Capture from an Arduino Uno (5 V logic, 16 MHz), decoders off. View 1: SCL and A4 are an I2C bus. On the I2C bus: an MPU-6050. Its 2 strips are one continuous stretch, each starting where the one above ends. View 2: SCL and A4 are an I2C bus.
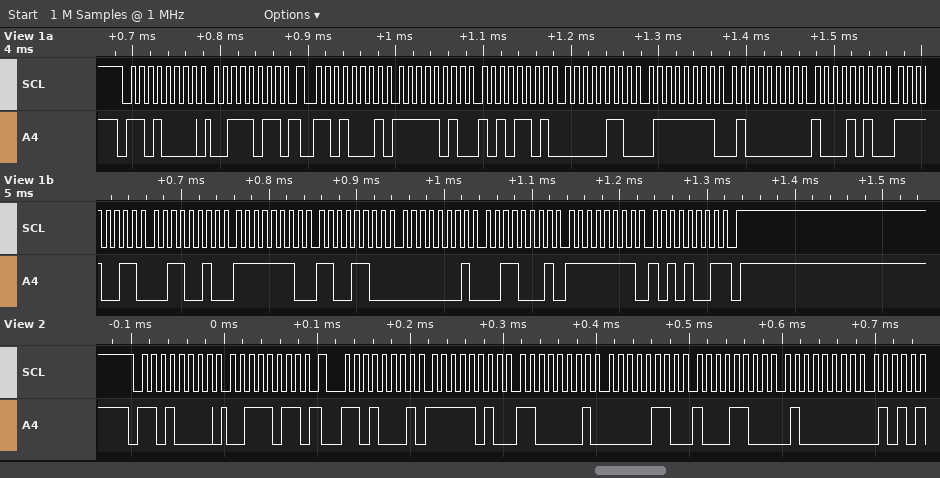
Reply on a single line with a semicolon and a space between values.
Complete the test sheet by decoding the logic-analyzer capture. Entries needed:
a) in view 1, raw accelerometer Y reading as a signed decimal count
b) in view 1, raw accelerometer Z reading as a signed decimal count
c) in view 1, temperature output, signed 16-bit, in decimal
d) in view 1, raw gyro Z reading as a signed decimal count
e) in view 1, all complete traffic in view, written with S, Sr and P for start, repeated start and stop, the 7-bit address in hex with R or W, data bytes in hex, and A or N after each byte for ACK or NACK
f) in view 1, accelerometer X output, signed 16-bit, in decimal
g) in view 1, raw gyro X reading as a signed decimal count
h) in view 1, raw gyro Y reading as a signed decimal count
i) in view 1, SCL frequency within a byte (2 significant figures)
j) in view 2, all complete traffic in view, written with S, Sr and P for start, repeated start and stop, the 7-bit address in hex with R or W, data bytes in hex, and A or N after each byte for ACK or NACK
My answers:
1663; 16522; -3278; -87; S 68W A 3B A Sr 68R A FA A AD A 06 A 7F A 40 A 8A A F3 A 32 A FE A CC A 01 A 31 A FF A A9 N P; -1363; -308; 305; 100 kHz; S 68W A 3B A Sr 68R A FA A C1 A 06 A 8C A 40 A
